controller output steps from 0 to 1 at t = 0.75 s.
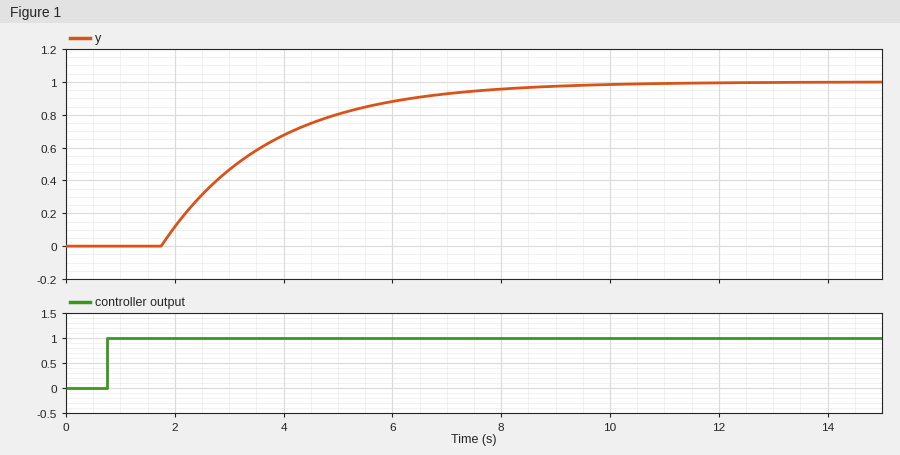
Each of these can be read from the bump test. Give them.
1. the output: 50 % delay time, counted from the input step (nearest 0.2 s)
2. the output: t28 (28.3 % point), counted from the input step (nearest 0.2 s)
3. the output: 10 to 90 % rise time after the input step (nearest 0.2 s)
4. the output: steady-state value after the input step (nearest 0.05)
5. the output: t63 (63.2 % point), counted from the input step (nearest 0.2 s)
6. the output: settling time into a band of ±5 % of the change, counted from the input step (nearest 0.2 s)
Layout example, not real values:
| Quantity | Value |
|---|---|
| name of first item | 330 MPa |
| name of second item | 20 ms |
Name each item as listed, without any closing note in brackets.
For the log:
| Quantity | Value |
|---|---|
| the output: 50 % delay time, counted from the input step | 2.4 s |
| the output: t28 (28.3 % point), counted from the input step | 1.6 s |
| the output: 10 to 90 % rise time after the input step | 4.4 s |
| the output: steady-state value after the input step | 1.00 |
| the output: t63 (63.2 % point), counted from the input step | 3.0 s |
| the output: settling time into a band of ±5 % of the change, counted from the input step | 7.0 s |
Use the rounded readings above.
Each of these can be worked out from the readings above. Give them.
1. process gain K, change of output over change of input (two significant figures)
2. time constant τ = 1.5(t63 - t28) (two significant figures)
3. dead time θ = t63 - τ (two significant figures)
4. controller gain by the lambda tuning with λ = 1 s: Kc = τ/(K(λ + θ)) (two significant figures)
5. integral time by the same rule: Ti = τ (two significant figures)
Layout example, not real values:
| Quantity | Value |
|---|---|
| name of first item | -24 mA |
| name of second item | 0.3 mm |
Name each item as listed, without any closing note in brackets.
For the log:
| Quantity | Value |
|---|---|
| process gain K, change of output over change of input | 1.0 |
| time constant τ = 1.5(t63 - t28) | 2.1 s |
| dead time θ = t63 - τ | 0.90 s |
| controller gain by the lambda tuning with λ = 1 s: Kc = τ/(K(λ + θ)) | 1.1 |
| integral time by the same rule: Ti = τ | 2.1 s |
